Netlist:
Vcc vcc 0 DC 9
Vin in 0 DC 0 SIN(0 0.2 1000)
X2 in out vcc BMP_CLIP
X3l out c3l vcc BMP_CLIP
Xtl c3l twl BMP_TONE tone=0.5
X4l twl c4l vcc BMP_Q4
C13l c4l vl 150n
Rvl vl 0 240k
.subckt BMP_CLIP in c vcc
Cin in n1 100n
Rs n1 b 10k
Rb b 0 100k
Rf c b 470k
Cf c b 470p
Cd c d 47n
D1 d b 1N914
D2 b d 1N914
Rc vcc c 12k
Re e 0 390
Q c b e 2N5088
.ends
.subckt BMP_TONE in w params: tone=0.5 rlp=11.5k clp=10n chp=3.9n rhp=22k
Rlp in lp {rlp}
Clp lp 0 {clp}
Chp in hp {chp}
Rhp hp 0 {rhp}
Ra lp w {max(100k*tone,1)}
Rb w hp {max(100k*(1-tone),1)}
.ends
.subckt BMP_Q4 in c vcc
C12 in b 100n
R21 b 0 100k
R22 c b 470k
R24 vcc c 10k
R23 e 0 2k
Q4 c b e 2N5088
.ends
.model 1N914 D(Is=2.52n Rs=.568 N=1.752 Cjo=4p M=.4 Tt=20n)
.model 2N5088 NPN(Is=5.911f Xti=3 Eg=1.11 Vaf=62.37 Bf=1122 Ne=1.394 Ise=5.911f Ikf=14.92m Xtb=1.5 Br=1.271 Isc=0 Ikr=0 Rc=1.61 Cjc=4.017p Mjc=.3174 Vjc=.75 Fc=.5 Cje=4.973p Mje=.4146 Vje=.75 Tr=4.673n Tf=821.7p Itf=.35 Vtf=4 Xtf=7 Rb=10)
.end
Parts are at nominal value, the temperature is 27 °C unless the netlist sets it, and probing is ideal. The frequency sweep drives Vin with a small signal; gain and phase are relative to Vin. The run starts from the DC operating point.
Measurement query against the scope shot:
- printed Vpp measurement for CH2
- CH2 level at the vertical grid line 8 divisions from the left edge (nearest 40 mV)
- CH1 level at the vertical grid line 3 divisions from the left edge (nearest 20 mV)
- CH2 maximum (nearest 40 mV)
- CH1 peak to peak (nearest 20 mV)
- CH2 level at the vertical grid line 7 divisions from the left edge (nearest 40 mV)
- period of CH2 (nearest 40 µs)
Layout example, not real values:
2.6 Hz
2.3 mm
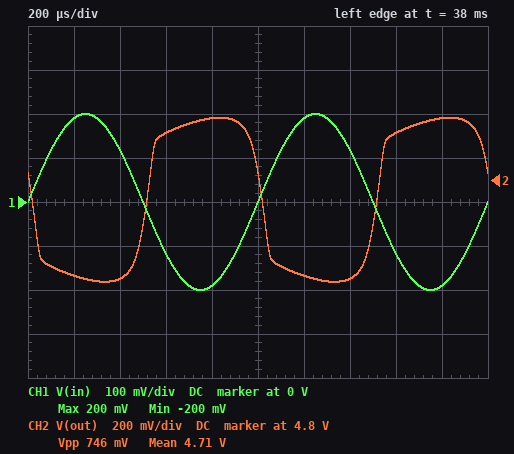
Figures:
746 mV
5.00 V
-120 mV
5.08 V
400 mV
4.36 V
1.00 ms
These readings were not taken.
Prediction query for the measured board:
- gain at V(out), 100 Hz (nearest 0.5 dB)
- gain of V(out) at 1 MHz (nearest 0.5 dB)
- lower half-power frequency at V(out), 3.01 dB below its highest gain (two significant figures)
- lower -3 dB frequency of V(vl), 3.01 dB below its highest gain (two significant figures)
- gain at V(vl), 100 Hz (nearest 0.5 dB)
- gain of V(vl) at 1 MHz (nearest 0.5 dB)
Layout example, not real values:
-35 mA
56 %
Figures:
20.0 dB
-26.0 dB
42 Hz
71 Hz
43.5 dB
-53.5 dB
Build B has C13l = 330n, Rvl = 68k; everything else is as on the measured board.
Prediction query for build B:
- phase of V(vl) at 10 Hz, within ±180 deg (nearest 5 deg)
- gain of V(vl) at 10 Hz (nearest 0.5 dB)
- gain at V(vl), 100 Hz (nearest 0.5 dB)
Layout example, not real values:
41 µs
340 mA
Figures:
75 deg
7.0 dB
43.0 dB
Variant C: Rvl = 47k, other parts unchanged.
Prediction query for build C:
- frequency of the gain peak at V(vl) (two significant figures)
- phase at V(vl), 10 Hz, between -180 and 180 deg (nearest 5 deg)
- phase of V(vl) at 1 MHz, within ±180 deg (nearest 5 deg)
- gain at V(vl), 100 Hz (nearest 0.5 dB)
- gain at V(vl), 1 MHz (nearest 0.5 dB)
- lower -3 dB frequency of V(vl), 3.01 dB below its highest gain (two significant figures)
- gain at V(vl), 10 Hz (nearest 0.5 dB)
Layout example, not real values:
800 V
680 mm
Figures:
230 Hz
105 deg
-160 deg
42.5 dB
-54.0 dB
73 Hz
1.0 dB
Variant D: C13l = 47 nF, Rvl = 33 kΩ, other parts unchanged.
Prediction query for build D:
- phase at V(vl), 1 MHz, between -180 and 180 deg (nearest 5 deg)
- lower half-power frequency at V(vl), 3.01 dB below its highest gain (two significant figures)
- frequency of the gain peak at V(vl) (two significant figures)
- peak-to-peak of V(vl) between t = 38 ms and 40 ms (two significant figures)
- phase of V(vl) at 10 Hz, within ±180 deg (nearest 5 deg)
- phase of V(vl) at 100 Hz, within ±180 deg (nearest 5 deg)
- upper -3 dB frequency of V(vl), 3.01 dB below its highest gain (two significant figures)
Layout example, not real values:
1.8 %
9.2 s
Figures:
-160 deg
100 Hz
280 Hz
970 mV
125 deg
-85 deg
840 Hz
